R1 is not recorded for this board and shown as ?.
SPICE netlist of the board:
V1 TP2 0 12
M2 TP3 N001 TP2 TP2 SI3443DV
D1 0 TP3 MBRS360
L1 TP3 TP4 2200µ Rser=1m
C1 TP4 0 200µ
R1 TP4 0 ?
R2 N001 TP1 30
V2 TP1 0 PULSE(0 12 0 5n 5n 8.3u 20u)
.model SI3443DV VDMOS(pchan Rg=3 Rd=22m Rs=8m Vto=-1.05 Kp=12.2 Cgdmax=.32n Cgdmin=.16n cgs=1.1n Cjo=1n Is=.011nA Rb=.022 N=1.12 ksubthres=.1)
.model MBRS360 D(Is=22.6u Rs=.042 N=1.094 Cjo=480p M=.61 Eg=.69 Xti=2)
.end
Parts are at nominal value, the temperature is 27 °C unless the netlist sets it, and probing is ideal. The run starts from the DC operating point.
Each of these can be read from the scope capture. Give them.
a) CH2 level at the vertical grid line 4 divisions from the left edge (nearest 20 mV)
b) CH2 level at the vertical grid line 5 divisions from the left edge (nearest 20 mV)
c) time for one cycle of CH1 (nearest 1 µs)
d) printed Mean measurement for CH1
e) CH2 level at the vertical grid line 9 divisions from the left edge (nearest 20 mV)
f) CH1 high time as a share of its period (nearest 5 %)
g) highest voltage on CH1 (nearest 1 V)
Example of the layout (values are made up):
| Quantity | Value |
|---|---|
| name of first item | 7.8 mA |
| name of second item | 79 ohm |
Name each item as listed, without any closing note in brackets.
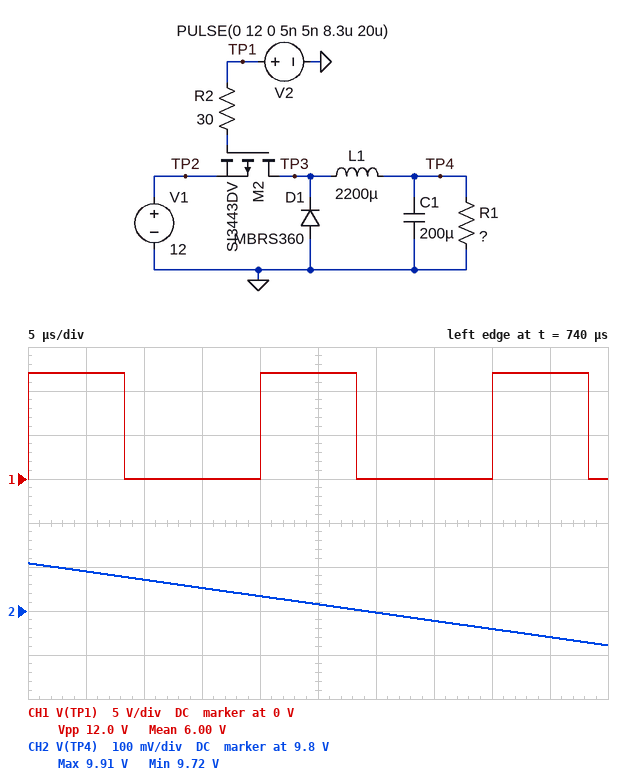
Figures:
| Quantity | Value |
|---|---|
| CH2 level at the vertical grid line 4 divisions from the left edge | 9.84 V |
| CH2 level at the vertical grid line 5 divisions from the left edge | 9.82 V |
| time for one cycle of CH1 | 20 µs |
| printed Mean measurement for CH1 | 6.00 V |
| CH2 level at the vertical grid line 9 divisions from the left edge | 9.74 V |
| CH1 high time as a share of its period | 40 % |
| highest voltage on CH1 | 12 V |
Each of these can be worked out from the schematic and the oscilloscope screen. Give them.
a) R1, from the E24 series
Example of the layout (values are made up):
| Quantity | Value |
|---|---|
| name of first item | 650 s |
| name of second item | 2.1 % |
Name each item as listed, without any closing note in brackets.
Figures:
| Quantity | Value |
|---|---|
| R1, from the E24 series | 2.7 Ω |
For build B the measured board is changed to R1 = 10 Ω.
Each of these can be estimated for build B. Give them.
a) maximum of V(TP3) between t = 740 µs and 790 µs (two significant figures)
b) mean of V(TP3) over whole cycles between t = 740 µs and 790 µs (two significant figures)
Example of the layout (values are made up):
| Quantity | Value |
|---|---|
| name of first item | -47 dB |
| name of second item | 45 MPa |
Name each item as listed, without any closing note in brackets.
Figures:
| Quantity | Value |
|---|---|
| maximum of V(TP3) between t = 740 µs and 790 µs | 13 V |
| mean of V(TP3) over whole cycles between t = 740 µs and 790 µs | 9.5 V |
